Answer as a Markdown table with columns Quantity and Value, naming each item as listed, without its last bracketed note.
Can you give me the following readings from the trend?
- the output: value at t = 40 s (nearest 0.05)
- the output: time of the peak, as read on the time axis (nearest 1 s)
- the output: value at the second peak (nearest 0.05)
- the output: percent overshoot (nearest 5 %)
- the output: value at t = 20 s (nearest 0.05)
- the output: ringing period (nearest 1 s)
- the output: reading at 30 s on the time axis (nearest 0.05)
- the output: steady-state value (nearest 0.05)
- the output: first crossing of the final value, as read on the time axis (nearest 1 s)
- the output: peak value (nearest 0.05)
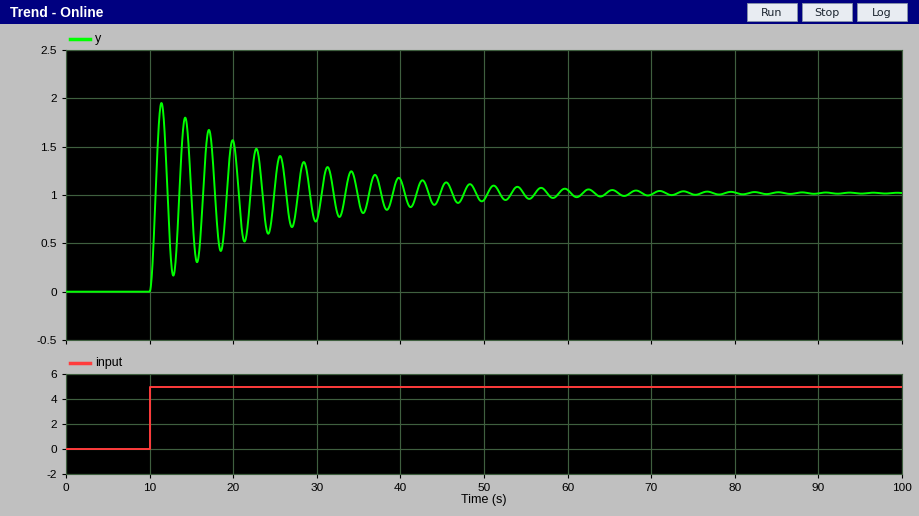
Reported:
| Quantity | Value |
|---|---|
| the output: value at t = 40 s | 1.15 |
| the output: time of the peak, as read on the time axis | 11 s |
| the output: value at the second peak | 1.80 |
| the output: percent overshoot | 90 % |
| the output: value at t = 20 s | 1.55 |
| the output: ringing period | 3 s |
| the output: reading at 30 s on the time axis | 0.75 |
| the output: steady-state value | 1.00 |
| the output: first crossing of the final value, as read on the time axis | 11 s |
| the output: peak value | 1.95 |
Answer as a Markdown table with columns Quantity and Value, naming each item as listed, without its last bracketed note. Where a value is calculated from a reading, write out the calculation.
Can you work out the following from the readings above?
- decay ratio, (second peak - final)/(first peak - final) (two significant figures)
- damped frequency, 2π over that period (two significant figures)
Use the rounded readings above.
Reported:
| Quantity | Value |
|---|---|
| decay ratio, (second peak - final)/(first peak - final) | (1.8 - 1) / (1.95 - 1) = 0.84 |
| damped frequency, 2π over that period | 2π / 3 = 2.1 rad/s |
